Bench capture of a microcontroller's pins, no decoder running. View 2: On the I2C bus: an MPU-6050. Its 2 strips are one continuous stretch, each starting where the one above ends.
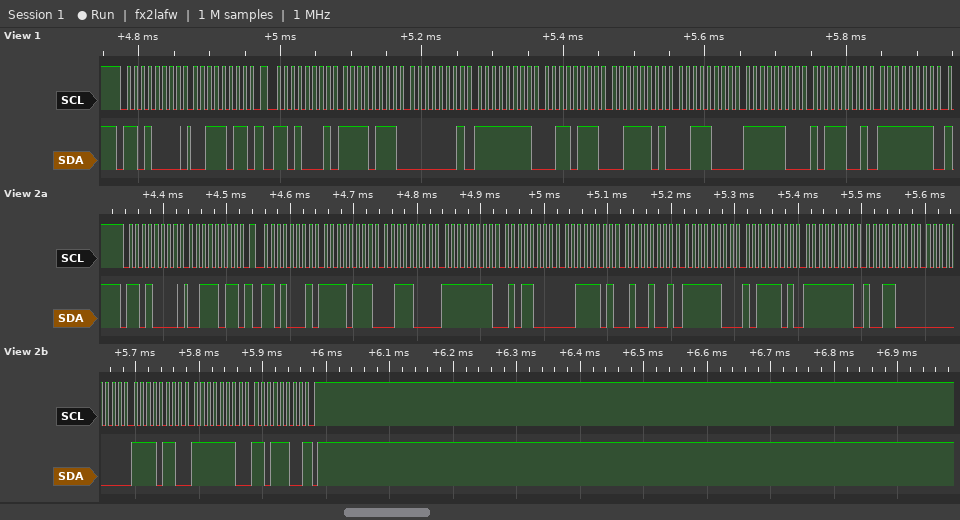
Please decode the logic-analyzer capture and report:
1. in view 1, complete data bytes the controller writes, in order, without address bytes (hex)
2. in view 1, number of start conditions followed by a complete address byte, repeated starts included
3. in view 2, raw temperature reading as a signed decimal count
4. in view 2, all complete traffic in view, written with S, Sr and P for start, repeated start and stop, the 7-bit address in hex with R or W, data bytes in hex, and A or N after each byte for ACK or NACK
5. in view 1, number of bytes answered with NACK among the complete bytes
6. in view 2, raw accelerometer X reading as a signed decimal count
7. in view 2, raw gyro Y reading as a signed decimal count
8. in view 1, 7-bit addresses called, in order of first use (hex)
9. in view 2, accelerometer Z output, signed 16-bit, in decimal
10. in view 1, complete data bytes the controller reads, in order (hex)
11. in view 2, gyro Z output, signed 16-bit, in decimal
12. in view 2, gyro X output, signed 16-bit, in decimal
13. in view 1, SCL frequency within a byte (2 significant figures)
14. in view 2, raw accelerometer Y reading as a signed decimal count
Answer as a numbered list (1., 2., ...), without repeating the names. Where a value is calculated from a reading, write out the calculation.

1. 3B
2. 2
3. 0xFCBD = -835
4. S 68W A 3B A Sr 68R A F7 A 38 A FF A 58 A 3D A 49 A FC A BD A FF A 98 A 00 A F6 A FE A DC N P
5. 0
6. 0xF738 = -2248
7. 0x00F6 = 246
8. 0x68
9. 0x3D49 = 15689
10. F7 01 FF 37 3D 38 FC B9 FF
11. 0xFEDC = -292
12. 0xFF98 = -104
13. 100 kHz
14. 0xFF58 = -168
